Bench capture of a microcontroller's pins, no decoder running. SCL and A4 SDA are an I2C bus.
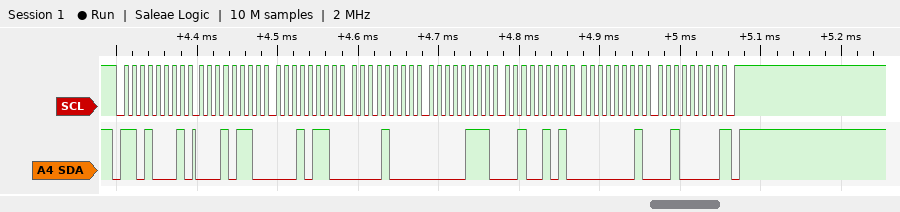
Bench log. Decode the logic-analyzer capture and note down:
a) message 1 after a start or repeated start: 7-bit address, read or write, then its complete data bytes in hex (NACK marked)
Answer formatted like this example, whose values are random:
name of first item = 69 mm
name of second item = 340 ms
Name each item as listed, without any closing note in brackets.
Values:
message 1 after a start or repeated start: 7-bit address, read or write, then its complete data bytes in hex = 0x68 read: 16 16 08 07 25 01 20 NACK
